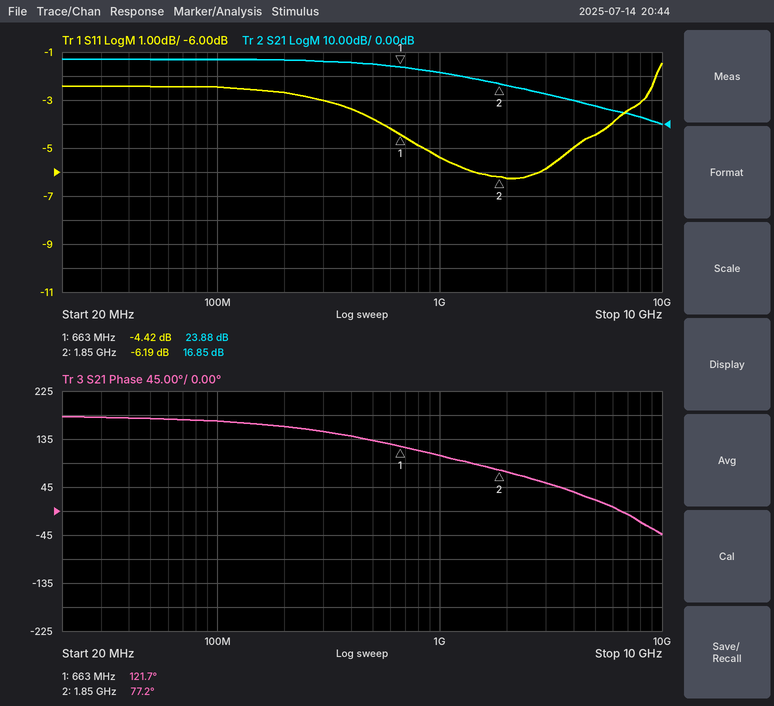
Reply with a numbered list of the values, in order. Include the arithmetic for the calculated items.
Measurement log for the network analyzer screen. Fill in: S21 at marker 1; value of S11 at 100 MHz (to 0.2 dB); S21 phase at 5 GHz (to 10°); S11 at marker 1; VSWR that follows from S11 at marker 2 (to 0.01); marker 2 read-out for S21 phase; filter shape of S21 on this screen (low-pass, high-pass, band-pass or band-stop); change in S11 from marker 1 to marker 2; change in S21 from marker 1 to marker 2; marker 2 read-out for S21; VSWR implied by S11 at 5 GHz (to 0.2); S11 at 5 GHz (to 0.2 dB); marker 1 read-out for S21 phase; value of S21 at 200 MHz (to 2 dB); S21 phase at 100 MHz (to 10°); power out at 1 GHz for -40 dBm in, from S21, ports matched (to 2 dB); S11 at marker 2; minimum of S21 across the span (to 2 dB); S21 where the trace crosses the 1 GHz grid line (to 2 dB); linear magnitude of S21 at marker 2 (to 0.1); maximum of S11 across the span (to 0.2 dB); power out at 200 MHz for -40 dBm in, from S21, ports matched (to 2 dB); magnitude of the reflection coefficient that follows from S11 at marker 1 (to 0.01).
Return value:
1. 23.88 dB
2. -2.4 dB
3. 20°
4. -4.42 dB
5. (1 + 0.4903)/(1 − 0.4903) ≈ 2.92
6. 77.2°
7. low-pass
8. -6.19 − (-4.42) = -1.77 dB
9. 16.85 − (23.88) = -7.03 dB
10. 16.85 dB
11. |Γ| = 10^(-4.4/20) = 0.6026; VSWR = (1 + 0.6026)/(1 − 0.6026) ≈ 4.0
12. -4.4 dB
13. 121.7°
14. 26 dB
15. 170°
16. -40 dBm + (22 dB) = -18 dBm
17. -6.19 dB
18. 0 dB
19. 22 dB
20. 10^(16.85/20) ≈ 7.0
21. -1.4 dB
22. -40 dBm + (26 dB) = -14 dBm
23. 10^(-4.42/20) ≈ 0.60
